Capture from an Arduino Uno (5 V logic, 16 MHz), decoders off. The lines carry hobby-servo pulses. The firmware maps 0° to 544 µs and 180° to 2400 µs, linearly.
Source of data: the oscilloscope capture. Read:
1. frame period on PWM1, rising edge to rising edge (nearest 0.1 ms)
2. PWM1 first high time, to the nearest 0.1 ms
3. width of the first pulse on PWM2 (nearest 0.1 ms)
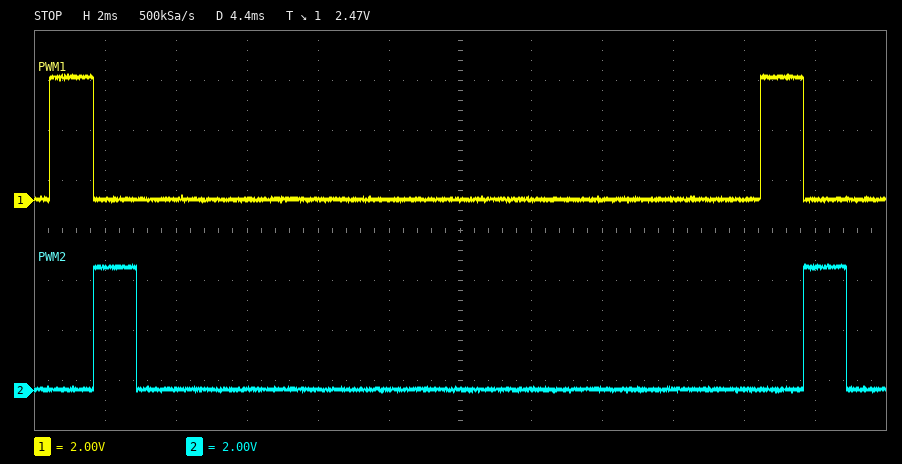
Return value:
20.0 ms
1.2 ms
1.2 ms
